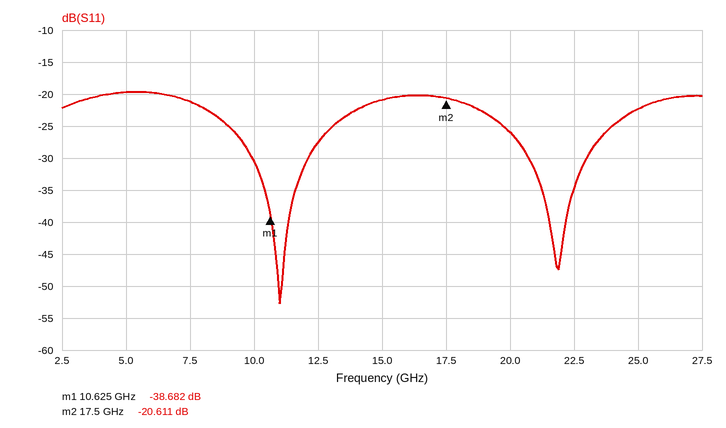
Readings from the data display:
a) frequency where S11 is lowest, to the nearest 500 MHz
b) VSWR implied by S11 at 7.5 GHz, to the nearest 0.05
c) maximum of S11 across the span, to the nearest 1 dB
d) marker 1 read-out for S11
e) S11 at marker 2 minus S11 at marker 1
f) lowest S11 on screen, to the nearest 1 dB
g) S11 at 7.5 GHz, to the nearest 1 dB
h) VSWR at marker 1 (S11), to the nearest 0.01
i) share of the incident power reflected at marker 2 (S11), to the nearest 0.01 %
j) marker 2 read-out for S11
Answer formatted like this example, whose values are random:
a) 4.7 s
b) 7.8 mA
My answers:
a) 11.0 GHz
b) 1.20
c) -20 dB
d) -38.682 dB
e) 18.071 dB
f) -53 dB
g) -21 dB
h) 1.02
i) 0.87 %
j) -20.611 dB
